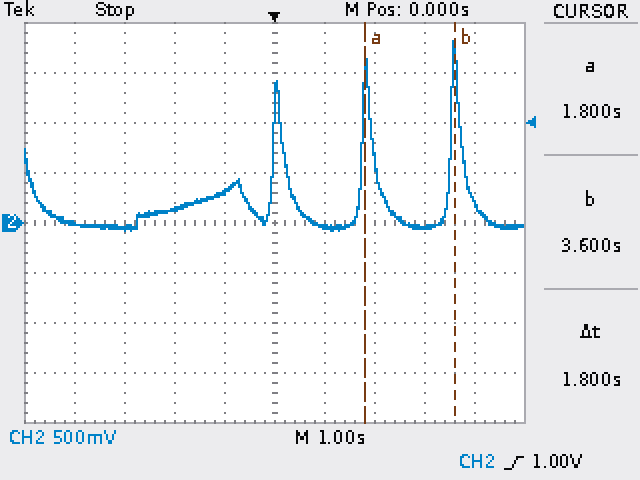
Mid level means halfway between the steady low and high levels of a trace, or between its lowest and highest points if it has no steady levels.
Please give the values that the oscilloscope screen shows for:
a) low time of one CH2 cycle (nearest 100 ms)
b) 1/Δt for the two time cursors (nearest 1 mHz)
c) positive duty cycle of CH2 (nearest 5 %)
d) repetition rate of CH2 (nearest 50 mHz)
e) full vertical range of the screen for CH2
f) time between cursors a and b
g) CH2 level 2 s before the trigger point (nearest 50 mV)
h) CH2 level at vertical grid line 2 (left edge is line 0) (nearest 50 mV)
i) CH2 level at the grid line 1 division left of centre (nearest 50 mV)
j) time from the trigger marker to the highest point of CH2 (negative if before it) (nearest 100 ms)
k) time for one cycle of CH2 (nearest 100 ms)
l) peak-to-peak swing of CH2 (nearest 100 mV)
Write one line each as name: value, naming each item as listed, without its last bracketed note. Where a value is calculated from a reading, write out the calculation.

low time of one CH2 cycle: 1.6 s
1/Δt for the two time cursors: 1 / 1.8 s ≈ 556 mHz
positive duty cycle of CH2: 10 %
repetition rate of CH2: 1 / 1.8 s ≈ 556 mHz, so 550 mHz to the nearest 50 mHz
full vertical range of the screen for CH2: 4 V
time between cursors a and b: 1.8 s
CH2 level 2 s before the trigger point: 150 mV
CH2 level at vertical grid line 2 (left edge is line 0): -50 mV
CH2 level at the grid line 1 division left of centre: 300 mV
time from the trigger marker to the highest point of CH2 (negative if before it): +3.6 s
time for one cycle of CH2: 1.8 s
peak-to-peak swing of CH2: 1.90 V
